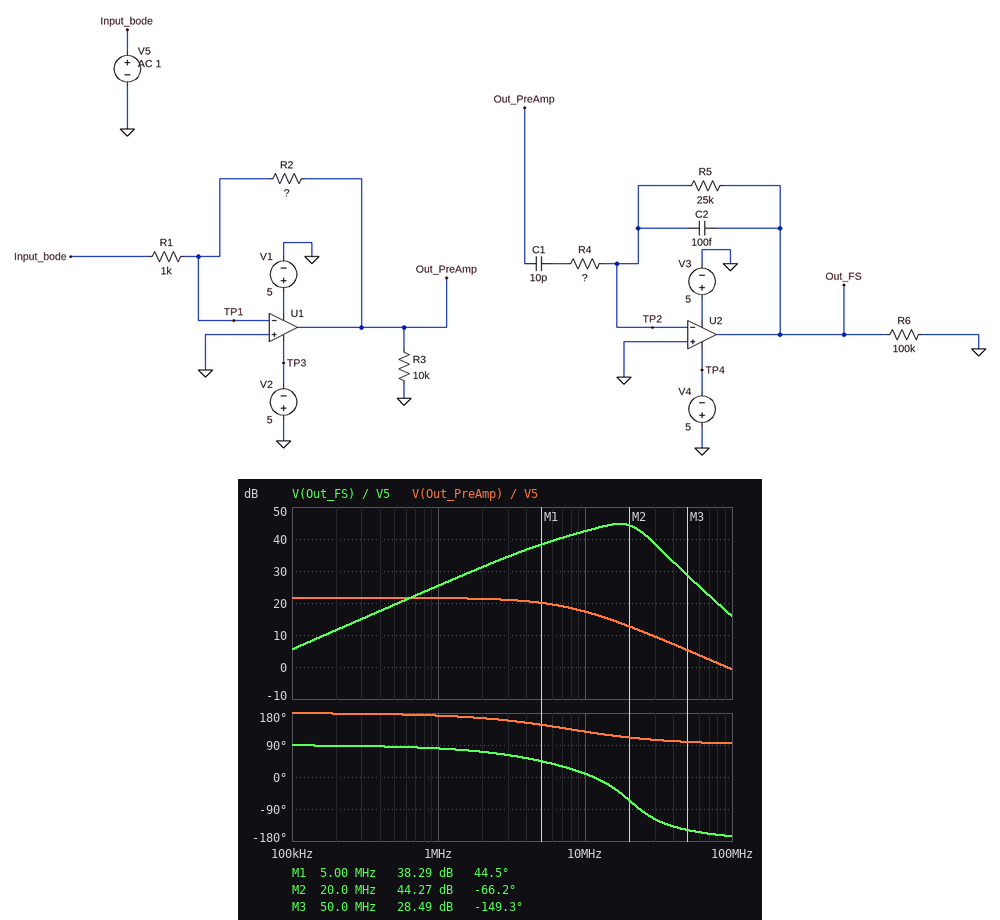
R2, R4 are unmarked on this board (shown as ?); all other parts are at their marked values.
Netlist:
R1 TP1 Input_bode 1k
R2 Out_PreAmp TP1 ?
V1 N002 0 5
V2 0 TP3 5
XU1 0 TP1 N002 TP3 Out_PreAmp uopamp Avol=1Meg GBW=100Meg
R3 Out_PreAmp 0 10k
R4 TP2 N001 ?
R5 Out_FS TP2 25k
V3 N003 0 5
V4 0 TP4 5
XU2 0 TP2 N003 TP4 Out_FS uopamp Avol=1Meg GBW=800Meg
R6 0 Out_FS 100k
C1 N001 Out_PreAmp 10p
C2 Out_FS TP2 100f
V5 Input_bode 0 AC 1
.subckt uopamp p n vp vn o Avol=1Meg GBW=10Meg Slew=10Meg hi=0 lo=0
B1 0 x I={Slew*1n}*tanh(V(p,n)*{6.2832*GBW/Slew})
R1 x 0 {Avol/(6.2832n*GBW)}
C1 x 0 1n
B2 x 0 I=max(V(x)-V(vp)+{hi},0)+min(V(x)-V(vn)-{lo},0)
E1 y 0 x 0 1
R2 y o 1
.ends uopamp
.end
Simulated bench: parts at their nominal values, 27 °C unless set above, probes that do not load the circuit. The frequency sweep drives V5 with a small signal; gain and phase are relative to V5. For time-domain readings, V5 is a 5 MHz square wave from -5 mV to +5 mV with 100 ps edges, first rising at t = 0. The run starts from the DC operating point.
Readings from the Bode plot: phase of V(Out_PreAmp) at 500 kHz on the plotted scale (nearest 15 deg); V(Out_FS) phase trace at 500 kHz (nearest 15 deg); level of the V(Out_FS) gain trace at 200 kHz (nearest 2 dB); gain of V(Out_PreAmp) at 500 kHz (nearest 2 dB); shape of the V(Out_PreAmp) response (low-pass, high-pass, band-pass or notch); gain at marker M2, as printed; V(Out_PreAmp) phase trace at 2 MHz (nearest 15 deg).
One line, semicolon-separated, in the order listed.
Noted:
180 deg; 90 deg; 12 dB; 22 dB; low-pass; 44.27 dB; 165 deg
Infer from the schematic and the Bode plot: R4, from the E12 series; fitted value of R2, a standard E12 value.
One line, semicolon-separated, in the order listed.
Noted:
390 Ω; 12 kΩ
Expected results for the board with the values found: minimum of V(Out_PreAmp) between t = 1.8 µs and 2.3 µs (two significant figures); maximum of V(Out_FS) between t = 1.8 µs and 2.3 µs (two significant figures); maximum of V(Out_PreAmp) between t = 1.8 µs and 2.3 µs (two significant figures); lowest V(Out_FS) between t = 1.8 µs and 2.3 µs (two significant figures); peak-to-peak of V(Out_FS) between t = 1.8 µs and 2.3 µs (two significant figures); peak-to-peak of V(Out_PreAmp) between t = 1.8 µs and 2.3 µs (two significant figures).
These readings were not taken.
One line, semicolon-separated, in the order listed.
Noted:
-59 mV; 500 mV; 59 mV; -500 mV; 1.0 V; 120 mV
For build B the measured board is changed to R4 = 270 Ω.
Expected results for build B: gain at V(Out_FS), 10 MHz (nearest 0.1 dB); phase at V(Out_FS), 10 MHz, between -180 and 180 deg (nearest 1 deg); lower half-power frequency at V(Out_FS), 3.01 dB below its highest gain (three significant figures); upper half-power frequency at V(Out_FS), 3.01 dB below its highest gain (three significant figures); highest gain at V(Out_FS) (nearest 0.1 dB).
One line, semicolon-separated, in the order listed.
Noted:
42.7 dB; 14 deg; 10.7 MHz; 25.4 MHz; 46.1 dB
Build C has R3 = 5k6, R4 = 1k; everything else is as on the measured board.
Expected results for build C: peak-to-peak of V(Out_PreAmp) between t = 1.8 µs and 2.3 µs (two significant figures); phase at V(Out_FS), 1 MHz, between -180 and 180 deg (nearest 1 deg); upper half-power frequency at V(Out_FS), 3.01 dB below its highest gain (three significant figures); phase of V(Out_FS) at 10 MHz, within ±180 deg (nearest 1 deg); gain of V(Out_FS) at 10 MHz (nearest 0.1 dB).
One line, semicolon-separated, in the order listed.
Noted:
120 mV; 78 deg; 21.5 MHz; -11 deg; 40.7 dB
